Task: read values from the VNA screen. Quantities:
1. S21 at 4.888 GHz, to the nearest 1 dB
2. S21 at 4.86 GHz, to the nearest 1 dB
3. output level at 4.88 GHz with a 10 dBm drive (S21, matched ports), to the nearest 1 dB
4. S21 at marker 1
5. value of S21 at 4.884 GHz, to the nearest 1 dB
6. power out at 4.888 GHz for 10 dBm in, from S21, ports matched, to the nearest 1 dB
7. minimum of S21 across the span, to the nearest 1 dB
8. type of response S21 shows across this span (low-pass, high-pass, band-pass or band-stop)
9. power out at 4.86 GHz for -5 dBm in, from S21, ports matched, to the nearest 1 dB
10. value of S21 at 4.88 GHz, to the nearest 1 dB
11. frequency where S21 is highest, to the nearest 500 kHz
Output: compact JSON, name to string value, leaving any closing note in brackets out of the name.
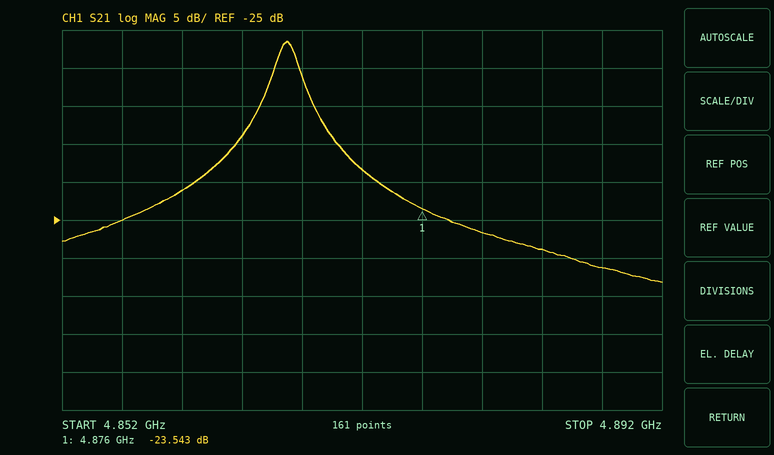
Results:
{"S21 at 4.888 GHz, to the nearest 1 dB": "-31 dB", "S21 at 4.86 GHz, to the nearest 1 dB": "-21 dB", "output level at 4.88 GHz with a 10 dBm drive (S21, matched ports), to the nearest 1 dB": "-17 dBm", "S21 at marker 1": "-23.543 dB", "value of S21 at 4.884 GHz, to the nearest 1 dB": "-29 dB", "power out at 4.888 GHz for 10 dBm in, from S21, ports matched, to the nearest 1 dB": "-21 dBm", "minimum of S21 across the span, to the nearest 1 dB": "-33 dB", "type of response S21 shows across this span": "band-pass", "power out at 4.86 GHz for -5 dBm in, from S21, ports matched, to the nearest 1 dB": "-26 dBm", "value of S21 at 4.88 GHz, to the nearest 1 dB": "-27 dB", "frequency where S21 is highest, to the nearest 500 kHz": "4.8670 GHz"}
